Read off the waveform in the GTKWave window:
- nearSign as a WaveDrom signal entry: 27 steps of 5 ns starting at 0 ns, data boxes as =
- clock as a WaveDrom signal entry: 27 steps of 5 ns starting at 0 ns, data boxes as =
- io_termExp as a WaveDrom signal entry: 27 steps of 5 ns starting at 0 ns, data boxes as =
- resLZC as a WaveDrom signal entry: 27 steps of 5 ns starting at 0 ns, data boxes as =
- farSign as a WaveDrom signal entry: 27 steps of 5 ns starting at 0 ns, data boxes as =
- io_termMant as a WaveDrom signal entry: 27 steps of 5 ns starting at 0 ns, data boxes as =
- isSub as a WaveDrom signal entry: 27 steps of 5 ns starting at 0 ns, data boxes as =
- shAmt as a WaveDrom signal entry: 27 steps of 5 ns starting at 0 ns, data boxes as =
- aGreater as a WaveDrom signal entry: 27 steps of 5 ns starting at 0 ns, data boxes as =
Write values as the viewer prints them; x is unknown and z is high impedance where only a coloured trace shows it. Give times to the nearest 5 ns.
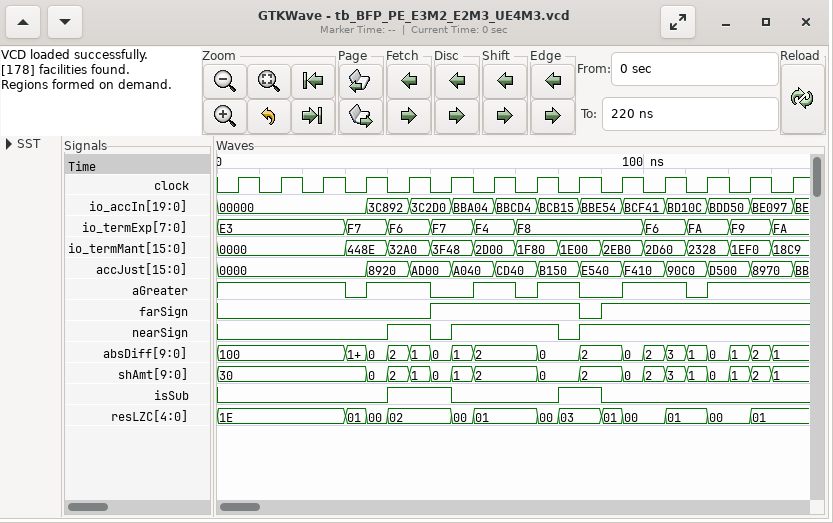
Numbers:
{name: 'nearSign', wave: '0.......1.01....01.........'}
{name: 'clock', wave: '010101010101010101010101010'}
{name: 'io_termExp', wave: '=.....=.=.=.=.=.....=.=.=.=', data: 'E3 F7 F6 F7 F4 F8 F6 FA F9 FA'}
{name: 'resLZC', wave: '=.....===..==..==.==.=.=.=.', data: '1E 01 00 02 00 01 00 03 01 00 01 00 01'}
{name: 'farSign', wave: '0.........1......01........'}
{name: 'io_termMant', wave: '=.....=.=.=.=.=.=.=.=.=.=.=', data: '0000 448E 32A0 3F48 2D00 1F80 1E00 2EB0 2D60 2328 1EF0 18C9'}
{name: 'isSub', wave: '0.......1..0....1.0........'}
{name: 'shAmt', wave: '=......======..=.=.========', data: '30 0 2 1 0 1 2 0 2 0 2 3 1 0 1 2 1'}
{name: 'aGreater', wave: '1.....01..0.1.01.0.1..01...'}
